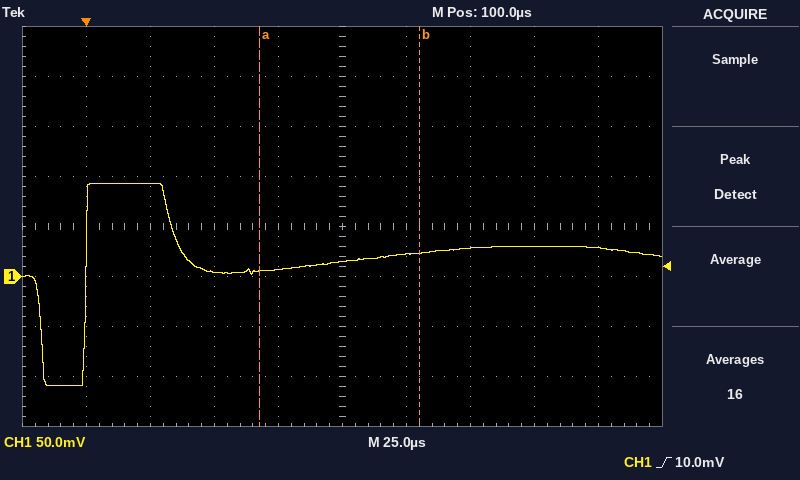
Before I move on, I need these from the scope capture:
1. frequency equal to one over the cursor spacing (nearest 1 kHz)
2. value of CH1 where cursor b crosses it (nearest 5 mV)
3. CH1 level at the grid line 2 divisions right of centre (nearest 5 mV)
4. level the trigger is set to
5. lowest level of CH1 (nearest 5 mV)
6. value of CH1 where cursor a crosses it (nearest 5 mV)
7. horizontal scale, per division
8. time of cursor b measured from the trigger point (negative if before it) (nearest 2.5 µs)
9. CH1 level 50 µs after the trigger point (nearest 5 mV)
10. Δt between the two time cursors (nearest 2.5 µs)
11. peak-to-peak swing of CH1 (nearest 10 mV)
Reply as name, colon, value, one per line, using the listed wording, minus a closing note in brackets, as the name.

frequency equal to one over the cursor spacing: 16 kHz
value of CH1 where cursor b crosses it: 25 mV
CH1 level at the grid line 2 divisions right of centre: 30 mV
level the trigger is set to: 10.0 mV
lowest level of CH1: -110 mV
value of CH1 where cursor a crosses it: 5 mV
horizontal scale, per division: 25 µs
time of cursor b measured from the trigger point (negative if before it): +130.0 µs
CH1 level 50 µs after the trigger point: 5 mV
Δt between the two time cursors: 62.5 µs
peak-to-peak swing of CH1: 200 mV
